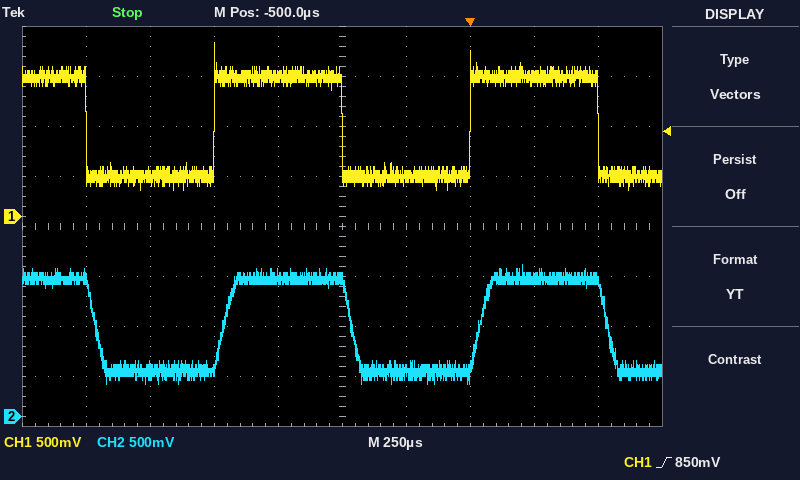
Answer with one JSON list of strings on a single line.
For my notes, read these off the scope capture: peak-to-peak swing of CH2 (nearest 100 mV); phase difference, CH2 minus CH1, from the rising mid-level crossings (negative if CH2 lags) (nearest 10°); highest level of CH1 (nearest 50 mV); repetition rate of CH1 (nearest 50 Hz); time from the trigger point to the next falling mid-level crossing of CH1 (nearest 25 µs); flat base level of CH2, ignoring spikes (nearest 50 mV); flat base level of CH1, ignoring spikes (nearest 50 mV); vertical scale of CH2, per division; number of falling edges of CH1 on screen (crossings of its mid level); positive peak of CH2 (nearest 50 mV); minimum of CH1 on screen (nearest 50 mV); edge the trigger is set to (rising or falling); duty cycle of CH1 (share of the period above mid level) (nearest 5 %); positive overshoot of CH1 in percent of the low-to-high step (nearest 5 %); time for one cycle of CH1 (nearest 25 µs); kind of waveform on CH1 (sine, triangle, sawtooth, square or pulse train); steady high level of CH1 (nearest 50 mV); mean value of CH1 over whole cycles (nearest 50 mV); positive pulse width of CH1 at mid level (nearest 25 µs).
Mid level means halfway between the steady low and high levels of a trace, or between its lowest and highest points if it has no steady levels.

["1.20 V", "-10°", "1.75 V", "1.00 kHz", "500 µs", "450 mV", "400 mV", "500 mV", "3", "1.50 V", "250 mV", "rising", "50 %", "35 %", "1.000 ms", "square", "1.40 V", "900 mV", "500 µs"]
